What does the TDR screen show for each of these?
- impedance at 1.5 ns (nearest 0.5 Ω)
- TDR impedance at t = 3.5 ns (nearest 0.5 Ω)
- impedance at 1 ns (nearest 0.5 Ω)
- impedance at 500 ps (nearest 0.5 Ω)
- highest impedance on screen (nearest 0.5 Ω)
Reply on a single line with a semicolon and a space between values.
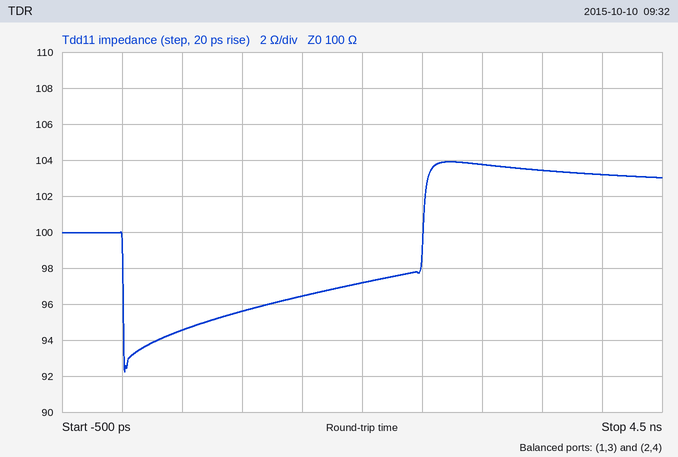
96.5 Ω; 103.5 Ω; 95.5 Ω; 94.5 Ω; 104.0 Ω
